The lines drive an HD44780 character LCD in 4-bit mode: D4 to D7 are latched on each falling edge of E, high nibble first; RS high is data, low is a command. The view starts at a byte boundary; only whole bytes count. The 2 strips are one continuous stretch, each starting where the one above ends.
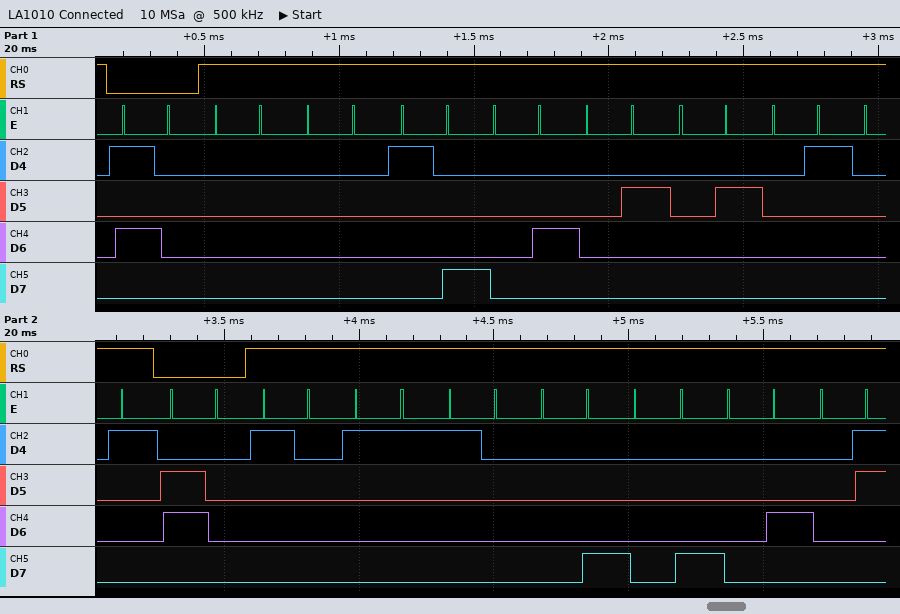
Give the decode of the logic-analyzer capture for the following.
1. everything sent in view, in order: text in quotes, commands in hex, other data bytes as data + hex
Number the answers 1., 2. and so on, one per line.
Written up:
1. 0x50 data 00 00 18 04 02 02 01 01 0x60 data 10 11 10 08 08 04 03
